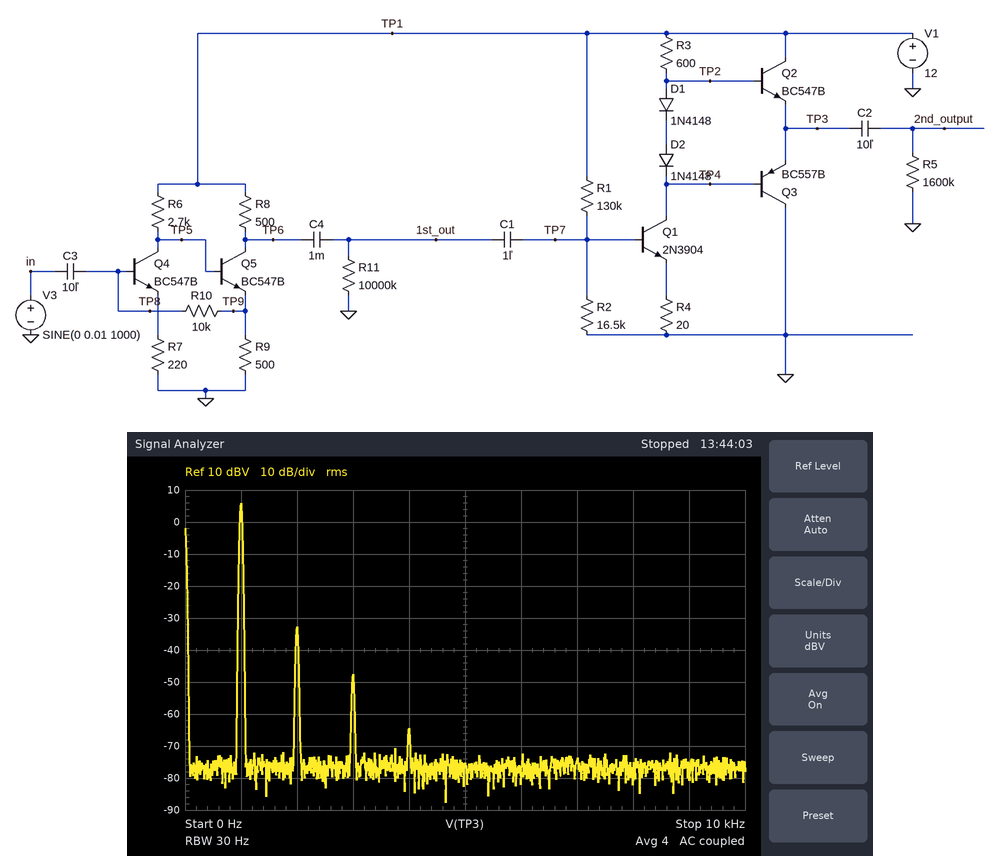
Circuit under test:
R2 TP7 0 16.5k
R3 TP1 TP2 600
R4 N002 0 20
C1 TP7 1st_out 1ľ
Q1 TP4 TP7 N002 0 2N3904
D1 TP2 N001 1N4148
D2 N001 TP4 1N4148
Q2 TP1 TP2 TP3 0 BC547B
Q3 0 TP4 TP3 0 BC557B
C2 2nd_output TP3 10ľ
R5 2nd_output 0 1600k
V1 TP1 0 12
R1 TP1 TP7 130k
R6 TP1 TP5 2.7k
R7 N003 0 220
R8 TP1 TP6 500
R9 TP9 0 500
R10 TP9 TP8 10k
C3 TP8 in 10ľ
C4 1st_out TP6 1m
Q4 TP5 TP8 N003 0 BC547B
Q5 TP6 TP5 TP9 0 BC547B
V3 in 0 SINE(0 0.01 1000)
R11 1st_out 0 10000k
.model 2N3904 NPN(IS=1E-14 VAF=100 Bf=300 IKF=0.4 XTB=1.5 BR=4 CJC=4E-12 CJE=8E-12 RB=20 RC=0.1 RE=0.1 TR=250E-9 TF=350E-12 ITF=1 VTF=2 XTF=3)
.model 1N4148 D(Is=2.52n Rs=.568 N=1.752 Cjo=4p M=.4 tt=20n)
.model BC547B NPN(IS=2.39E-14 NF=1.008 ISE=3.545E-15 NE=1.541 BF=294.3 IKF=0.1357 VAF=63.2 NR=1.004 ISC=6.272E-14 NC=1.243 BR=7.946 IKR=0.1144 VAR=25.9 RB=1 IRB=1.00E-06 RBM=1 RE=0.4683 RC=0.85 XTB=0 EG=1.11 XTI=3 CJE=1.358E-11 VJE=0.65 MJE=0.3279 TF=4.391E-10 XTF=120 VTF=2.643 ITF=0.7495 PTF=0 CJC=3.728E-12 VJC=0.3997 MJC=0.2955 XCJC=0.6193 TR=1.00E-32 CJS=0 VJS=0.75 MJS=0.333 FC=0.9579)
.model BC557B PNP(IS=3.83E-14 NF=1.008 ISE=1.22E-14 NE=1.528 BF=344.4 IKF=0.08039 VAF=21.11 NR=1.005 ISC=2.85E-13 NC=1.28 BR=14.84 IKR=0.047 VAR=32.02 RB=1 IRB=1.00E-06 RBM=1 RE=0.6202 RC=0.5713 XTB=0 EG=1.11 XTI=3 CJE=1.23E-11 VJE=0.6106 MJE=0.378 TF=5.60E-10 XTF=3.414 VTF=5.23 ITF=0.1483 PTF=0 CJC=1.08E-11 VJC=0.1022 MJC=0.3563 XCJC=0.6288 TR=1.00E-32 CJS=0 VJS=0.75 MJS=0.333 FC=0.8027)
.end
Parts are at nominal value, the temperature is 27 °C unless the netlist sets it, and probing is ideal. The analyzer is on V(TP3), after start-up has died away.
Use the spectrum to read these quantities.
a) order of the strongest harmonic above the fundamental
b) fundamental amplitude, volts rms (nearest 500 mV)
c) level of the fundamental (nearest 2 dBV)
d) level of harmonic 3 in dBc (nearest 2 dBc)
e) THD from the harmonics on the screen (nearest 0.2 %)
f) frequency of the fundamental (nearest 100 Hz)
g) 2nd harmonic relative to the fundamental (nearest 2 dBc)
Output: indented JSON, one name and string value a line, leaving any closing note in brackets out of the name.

{
  "order of the strongest harmonic above the fundamental": "2",
  "fundamental amplitude, volts rms": "2.0 V",
  "level of the fundamental": "6 dBV",
  "level of harmonic 3 in dBc": "-54 dBc",
  "THD from the harmonics on the screen": "1.2 %",
  "frequency of the fundamental": "1.0 kHz",
  "2nd harmonic relative to the fundamental": "-38 dBc"
}
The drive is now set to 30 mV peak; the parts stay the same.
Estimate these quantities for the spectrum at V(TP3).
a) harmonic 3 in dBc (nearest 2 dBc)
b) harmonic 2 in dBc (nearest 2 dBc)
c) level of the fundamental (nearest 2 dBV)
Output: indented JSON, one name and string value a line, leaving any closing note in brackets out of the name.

{
  "harmonic 3 in dBc": "-16 dBc",
  "harmonic 2 in dBc": "-24 dBc",
  "level of the fundamental": "12 dBV"
}
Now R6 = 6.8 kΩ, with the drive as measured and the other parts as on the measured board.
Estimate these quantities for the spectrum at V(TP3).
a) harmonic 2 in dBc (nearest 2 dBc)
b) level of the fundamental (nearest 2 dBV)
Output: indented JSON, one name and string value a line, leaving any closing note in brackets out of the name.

{
  "harmonic 2 in dBc": "-28 dBc",
  "level of the fundamental": "12 dBV"
}
